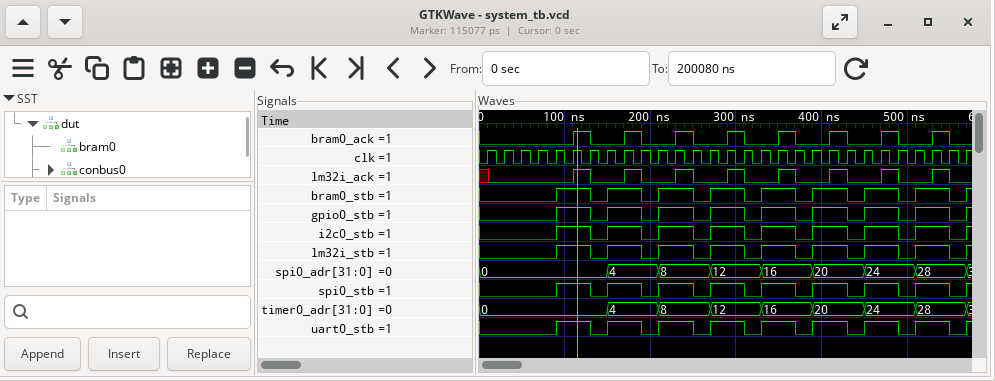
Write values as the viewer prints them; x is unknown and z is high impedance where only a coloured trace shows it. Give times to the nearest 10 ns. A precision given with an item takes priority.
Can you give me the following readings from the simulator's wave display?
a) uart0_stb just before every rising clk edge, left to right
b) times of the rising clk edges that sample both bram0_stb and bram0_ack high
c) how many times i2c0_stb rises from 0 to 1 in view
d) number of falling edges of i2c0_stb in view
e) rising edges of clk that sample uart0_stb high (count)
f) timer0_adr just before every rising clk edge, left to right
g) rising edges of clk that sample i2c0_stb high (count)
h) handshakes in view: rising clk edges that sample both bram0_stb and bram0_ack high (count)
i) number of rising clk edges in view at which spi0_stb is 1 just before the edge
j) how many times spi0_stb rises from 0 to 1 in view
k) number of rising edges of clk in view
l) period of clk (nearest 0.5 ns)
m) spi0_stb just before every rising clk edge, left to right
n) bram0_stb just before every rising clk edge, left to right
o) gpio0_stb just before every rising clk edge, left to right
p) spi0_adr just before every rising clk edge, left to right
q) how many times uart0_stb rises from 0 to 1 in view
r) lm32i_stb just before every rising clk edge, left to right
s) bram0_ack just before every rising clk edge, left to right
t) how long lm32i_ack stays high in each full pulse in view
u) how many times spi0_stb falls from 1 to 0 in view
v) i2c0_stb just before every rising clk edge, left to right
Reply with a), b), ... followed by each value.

a) 0 0 0 0 0 1 1 0 1 1 0 1 1 0 1 1 0 1 1 0 1 1 0 1 1 0 1 1 0
b) 130 ns, 190 ns, 250 ns, 310 ns, 370 ns, 430 ns, 490 ns, 550 ns
c) 9
d) 8
e) 16
f) 0, 0, 0, 0, 0, 0, 0, 0, 4, 4, 4, 8, 8, 8, 12, 12, 12, 16, 16, 16, 20, 20, 20, 24, 24, 24, 28, 28, 28
g) 16
h) 8
i) 16
j) 9
k) 29
l) 20 ns
m) 0 0 0 0 0 1 1 0 1 1 0 1 1 0 1 1 0 1 1 0 1 1 0 1 1 0 1 1 0
n) 0 0 0 0 0 1 1 0 1 1 0 1 1 0 1 1 0 1 1 0 1 1 0 1 1 0 1 1 0
o) 0 0 0 0 0 1 1 0 1 1 0 1 1 0 1 1 0 1 1 0 1 1 0 1 1 0 1 1 0
p) 0, 0, 0, 0, 0, 0, 0, 0, 4, 4, 4, 8, 8, 8, 12, 12, 12, 16, 16, 16, 20, 20, 20, 24, 24, 24, 28, 28, 28
q) 9
r) 0 0 0 0 0 1 1 0 1 1 0 1 1 0 1 1 0 1 1 0 1 1 0 1 1 0 1 1 0
s) 0 0 0 0 0 0 1 0 0 1 0 0 1 0 0 1 0 0 1 0 0 1 0 0 1 0 0 1 0
t) 20 ns, 20 ns, 20 ns, 20 ns, 20 ns, 20 ns, 20 ns, 20 ns
u) 8
v) 0 0 0 0 0 1 1 0 1 1 0 1 1 0 1 1 0 1 1 0 1 1 0 1 1 0 1 1 0
